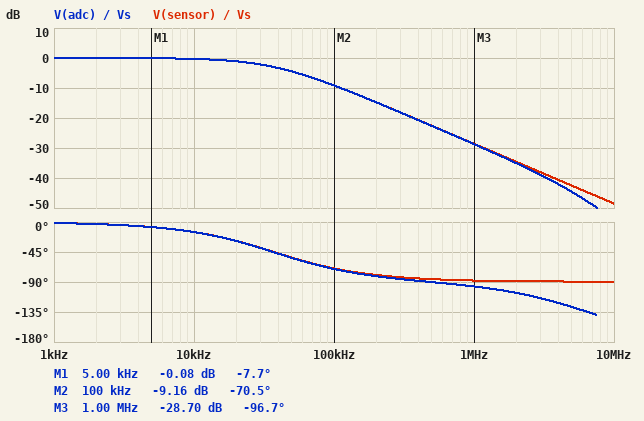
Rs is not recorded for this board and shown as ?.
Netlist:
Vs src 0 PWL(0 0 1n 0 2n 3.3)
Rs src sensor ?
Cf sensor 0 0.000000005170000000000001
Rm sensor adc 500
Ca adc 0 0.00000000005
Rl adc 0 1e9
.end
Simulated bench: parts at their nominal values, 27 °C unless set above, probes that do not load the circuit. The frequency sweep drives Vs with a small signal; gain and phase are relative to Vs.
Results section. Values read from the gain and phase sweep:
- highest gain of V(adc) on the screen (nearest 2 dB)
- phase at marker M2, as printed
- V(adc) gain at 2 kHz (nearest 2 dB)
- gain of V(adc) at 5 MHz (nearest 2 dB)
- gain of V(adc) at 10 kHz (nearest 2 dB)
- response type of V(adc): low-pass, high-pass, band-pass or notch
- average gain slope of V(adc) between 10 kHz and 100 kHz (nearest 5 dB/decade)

0 dB
-70.5 deg
0 dB
-44 dB
0 dB
low-pass
-10 dB/decade
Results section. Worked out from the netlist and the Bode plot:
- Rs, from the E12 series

820 Ω
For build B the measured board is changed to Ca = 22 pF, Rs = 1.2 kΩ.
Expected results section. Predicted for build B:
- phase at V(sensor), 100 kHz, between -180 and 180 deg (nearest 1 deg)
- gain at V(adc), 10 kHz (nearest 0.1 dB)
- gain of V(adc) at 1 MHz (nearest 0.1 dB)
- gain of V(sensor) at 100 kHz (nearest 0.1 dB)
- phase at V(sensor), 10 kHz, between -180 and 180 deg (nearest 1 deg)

-76 deg
-0.6 dB
-31.9 dB
-12.1 dB
-21 deg
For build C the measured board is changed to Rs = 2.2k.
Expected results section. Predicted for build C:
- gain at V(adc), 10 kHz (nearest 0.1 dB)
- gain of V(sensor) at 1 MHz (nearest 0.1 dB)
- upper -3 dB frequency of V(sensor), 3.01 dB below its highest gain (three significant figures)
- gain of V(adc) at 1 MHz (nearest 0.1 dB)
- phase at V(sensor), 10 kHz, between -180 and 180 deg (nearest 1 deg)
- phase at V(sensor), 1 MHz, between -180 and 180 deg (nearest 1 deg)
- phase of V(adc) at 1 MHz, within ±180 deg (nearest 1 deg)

-1.8 dB
-37.2 dB
13.9 kHz
-37.3 dB
-36 deg
-89 deg
-98 deg
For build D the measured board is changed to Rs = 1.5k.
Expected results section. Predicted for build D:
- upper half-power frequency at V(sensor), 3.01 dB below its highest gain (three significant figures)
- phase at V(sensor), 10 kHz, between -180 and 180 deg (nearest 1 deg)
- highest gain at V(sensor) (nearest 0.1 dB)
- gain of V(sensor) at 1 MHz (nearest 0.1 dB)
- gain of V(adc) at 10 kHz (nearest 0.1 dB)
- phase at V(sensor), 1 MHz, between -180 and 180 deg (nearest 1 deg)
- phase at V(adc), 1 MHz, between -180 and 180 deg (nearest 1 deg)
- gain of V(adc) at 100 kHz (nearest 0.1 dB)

20.3 kHz
-26 deg
0 dB
-33.8 dB
-0.9 dB
-89 deg
-98 deg
-14.0 dB
